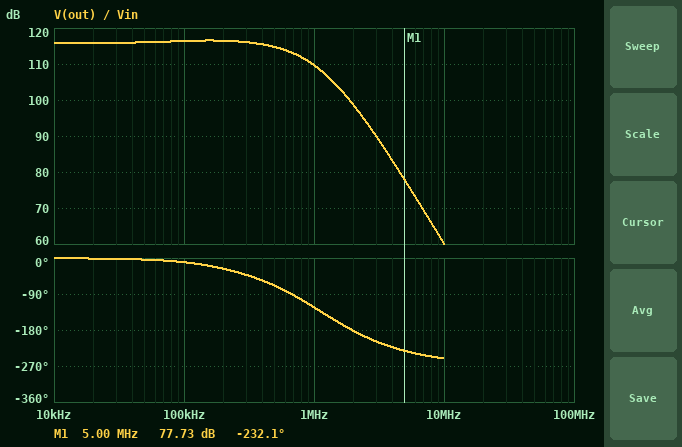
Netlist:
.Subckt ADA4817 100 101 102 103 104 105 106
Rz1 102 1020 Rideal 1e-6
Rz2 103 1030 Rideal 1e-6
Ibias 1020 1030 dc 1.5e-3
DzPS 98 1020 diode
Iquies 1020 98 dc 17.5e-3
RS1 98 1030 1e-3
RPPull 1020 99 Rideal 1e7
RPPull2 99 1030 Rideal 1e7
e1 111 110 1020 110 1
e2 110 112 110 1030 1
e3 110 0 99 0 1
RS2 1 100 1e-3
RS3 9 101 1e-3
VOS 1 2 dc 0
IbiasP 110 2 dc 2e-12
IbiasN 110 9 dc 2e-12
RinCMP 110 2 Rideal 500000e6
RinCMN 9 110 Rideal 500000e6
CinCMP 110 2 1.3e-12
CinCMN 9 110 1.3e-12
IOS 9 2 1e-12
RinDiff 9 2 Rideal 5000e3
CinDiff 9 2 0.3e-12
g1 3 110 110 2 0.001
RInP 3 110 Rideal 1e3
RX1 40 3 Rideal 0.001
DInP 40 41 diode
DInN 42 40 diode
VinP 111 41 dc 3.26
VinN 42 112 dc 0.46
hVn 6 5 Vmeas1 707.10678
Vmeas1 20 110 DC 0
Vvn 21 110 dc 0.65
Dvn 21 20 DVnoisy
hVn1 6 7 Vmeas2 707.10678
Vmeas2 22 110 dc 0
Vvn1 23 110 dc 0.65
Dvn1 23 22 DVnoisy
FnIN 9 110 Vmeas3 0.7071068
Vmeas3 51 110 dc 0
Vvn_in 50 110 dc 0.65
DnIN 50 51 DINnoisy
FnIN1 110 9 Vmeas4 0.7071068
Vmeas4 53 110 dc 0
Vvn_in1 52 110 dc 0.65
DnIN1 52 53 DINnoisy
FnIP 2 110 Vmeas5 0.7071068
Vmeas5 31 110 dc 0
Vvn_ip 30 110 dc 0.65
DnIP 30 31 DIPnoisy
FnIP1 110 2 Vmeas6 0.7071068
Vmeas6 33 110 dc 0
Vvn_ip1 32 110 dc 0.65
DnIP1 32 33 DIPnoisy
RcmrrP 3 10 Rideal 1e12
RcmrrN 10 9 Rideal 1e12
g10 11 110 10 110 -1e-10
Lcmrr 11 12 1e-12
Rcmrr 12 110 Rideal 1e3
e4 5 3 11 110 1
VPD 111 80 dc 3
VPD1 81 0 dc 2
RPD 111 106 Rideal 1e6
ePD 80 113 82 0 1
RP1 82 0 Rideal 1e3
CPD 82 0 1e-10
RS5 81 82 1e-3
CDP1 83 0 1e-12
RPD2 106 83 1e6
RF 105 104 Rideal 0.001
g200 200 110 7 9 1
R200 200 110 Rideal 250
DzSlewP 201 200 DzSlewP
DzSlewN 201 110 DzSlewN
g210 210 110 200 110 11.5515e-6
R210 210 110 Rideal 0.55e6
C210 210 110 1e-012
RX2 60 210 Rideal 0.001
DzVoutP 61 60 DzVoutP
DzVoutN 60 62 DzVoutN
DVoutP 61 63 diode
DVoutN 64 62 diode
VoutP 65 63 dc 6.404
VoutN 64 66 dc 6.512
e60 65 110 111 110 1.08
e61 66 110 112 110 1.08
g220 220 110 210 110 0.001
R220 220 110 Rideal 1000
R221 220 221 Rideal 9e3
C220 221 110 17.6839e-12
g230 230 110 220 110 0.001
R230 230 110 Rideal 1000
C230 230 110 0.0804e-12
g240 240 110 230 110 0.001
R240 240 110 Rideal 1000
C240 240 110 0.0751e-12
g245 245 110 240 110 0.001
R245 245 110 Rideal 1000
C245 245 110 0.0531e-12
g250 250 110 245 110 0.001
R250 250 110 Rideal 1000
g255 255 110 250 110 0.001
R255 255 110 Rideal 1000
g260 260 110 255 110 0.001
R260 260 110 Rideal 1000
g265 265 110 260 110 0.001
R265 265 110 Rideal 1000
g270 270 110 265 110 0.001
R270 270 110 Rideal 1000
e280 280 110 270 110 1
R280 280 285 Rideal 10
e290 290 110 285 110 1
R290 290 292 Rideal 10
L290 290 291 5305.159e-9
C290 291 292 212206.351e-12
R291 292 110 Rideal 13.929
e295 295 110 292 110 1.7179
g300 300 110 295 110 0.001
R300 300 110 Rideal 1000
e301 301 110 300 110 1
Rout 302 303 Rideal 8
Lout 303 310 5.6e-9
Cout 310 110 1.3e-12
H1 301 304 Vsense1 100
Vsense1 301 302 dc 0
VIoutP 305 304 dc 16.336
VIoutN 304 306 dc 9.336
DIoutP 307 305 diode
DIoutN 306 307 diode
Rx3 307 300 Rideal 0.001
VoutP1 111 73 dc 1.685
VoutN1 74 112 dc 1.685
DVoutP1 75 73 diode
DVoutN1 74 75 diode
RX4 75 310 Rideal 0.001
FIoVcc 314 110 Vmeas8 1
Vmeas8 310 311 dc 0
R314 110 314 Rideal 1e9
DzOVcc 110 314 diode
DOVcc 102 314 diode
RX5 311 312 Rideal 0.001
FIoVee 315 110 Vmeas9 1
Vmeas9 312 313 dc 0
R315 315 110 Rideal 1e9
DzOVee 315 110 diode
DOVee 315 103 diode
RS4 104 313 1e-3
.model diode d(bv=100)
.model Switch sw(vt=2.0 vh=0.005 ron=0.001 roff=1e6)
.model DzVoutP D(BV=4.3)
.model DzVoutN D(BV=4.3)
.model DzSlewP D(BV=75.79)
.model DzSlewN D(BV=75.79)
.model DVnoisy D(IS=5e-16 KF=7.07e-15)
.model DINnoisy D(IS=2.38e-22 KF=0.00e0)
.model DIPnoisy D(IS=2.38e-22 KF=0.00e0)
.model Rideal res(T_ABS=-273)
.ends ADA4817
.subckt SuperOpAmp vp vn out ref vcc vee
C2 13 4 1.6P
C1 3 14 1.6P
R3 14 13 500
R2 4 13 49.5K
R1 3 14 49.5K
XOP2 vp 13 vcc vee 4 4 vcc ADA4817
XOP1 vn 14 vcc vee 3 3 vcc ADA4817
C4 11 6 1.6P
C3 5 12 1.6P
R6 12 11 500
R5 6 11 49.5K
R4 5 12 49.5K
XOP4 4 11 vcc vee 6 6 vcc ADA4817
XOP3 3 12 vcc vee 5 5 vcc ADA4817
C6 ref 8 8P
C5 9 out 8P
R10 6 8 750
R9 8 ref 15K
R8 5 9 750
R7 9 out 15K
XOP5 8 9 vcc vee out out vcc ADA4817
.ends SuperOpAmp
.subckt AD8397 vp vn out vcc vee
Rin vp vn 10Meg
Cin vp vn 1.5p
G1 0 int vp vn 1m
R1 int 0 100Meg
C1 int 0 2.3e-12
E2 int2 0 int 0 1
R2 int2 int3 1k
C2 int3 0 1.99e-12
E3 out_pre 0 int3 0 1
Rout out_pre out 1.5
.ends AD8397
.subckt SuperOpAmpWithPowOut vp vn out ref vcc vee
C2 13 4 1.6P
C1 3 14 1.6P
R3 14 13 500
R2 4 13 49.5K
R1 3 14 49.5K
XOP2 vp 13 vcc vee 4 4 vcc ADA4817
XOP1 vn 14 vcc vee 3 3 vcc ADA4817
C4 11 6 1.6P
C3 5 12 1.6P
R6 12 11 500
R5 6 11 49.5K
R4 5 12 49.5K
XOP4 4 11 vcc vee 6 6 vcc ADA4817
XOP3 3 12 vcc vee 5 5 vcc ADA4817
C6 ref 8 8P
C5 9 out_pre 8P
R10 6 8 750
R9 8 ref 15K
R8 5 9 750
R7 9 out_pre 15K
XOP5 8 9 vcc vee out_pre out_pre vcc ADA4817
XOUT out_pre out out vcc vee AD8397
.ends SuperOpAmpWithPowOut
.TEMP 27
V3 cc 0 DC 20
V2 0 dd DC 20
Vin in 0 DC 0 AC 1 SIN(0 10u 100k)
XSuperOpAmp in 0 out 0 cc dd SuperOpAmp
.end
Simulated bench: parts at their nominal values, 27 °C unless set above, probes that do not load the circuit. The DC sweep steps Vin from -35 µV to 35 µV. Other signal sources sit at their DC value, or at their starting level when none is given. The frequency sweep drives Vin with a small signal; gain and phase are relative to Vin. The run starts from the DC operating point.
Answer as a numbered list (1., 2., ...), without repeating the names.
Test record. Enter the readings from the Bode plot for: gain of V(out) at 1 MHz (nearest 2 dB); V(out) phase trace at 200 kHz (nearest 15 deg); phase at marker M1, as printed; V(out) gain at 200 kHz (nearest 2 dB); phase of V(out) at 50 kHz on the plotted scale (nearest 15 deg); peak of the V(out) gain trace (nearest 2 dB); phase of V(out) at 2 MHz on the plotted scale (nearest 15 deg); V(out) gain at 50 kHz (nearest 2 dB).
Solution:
1. 110 dB
2. -30 deg
3. -232.1 deg
4. 116 dB
5. 0 deg
6. 116 dB
7. -180 deg
8. 116 dB
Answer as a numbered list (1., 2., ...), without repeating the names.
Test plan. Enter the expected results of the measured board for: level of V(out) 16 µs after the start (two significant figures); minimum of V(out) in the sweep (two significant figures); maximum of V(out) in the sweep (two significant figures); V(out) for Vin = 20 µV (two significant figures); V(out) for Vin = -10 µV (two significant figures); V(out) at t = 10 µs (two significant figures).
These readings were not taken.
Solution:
1. -2.8 V
2. -19 V
3. 19 V
4. 12 V
5. -6.2 V
6. -1.2 V
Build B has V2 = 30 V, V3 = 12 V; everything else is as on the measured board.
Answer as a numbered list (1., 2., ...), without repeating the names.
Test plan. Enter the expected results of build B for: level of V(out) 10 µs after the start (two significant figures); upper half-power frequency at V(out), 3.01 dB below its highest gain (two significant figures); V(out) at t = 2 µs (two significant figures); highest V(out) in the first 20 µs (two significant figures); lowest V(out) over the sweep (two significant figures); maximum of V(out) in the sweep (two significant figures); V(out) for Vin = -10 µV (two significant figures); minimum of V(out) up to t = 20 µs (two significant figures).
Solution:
1. -1.3 V
2. 640 kHz
3. 5.5 V
4. 6.5 V
5. -22 V
6. 11 V
7. -6.3 V
8. -6.7 V
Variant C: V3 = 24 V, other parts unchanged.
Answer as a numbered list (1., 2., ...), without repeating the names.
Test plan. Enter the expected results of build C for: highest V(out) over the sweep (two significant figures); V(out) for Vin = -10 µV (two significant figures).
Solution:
1. 22 V
2. -6.1 V
